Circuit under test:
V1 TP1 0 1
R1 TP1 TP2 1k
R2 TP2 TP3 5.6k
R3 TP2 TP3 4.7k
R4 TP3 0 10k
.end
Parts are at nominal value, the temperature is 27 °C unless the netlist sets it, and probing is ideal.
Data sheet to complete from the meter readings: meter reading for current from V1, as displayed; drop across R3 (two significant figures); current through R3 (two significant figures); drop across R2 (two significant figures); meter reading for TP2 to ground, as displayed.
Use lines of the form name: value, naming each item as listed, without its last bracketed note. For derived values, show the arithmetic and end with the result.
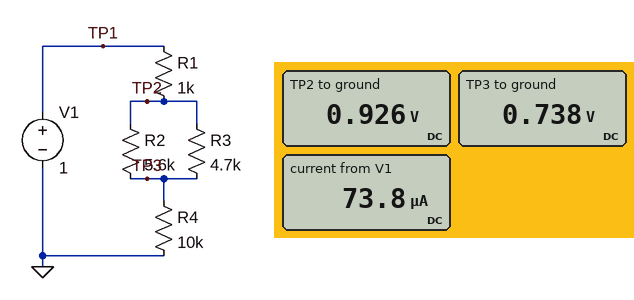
meter reading for current from V1, as displayed: 73.8 µA
drop across R3: 926 mV - 738 mV = 190 mV
current through R3: (926 mV - 738 mV) / 4.7 kΩ = 40 µA
drop across R2: 926 mV - 738 mV = 190 mV
meter reading for TP2 to ground, as displayed: 0.926 V
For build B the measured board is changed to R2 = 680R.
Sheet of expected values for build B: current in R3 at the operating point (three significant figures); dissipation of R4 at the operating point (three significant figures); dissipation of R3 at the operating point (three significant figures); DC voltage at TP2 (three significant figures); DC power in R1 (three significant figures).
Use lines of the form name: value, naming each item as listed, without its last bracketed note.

current in R3 at the operating point: 10.9 µA
dissipation of R4 at the operating point: 74.4 µW
dissipation of R3 at the operating point: 559 nW
DC voltage at TP2: 914 mV
DC power in R1: 7.44 µW
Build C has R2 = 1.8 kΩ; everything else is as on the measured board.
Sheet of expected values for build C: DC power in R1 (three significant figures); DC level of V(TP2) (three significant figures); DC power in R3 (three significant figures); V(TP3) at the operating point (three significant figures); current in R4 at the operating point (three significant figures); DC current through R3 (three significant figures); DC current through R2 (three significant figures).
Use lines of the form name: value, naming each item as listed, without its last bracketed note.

DC power in R1: 6.61 µW
DC level of V(TP2): 919 mV
DC power in R3: 2.38 µW
V(TP3) at the operating point: 813 mV
current in R4 at the operating point: 81.3 µA
DC current through R3: 22.5 µA
DC current through R2: 58.8 µA
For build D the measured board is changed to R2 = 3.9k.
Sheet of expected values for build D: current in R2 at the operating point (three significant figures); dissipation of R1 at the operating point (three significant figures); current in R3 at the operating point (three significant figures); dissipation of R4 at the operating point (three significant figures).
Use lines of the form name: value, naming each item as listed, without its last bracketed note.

current in R2 at the operating point: 41.6 µA
dissipation of R1 at the operating point: 5.80 µW
current in R3 at the operating point: 34.5 µA
dissipation of R4 at the operating point: 58.0 µW
